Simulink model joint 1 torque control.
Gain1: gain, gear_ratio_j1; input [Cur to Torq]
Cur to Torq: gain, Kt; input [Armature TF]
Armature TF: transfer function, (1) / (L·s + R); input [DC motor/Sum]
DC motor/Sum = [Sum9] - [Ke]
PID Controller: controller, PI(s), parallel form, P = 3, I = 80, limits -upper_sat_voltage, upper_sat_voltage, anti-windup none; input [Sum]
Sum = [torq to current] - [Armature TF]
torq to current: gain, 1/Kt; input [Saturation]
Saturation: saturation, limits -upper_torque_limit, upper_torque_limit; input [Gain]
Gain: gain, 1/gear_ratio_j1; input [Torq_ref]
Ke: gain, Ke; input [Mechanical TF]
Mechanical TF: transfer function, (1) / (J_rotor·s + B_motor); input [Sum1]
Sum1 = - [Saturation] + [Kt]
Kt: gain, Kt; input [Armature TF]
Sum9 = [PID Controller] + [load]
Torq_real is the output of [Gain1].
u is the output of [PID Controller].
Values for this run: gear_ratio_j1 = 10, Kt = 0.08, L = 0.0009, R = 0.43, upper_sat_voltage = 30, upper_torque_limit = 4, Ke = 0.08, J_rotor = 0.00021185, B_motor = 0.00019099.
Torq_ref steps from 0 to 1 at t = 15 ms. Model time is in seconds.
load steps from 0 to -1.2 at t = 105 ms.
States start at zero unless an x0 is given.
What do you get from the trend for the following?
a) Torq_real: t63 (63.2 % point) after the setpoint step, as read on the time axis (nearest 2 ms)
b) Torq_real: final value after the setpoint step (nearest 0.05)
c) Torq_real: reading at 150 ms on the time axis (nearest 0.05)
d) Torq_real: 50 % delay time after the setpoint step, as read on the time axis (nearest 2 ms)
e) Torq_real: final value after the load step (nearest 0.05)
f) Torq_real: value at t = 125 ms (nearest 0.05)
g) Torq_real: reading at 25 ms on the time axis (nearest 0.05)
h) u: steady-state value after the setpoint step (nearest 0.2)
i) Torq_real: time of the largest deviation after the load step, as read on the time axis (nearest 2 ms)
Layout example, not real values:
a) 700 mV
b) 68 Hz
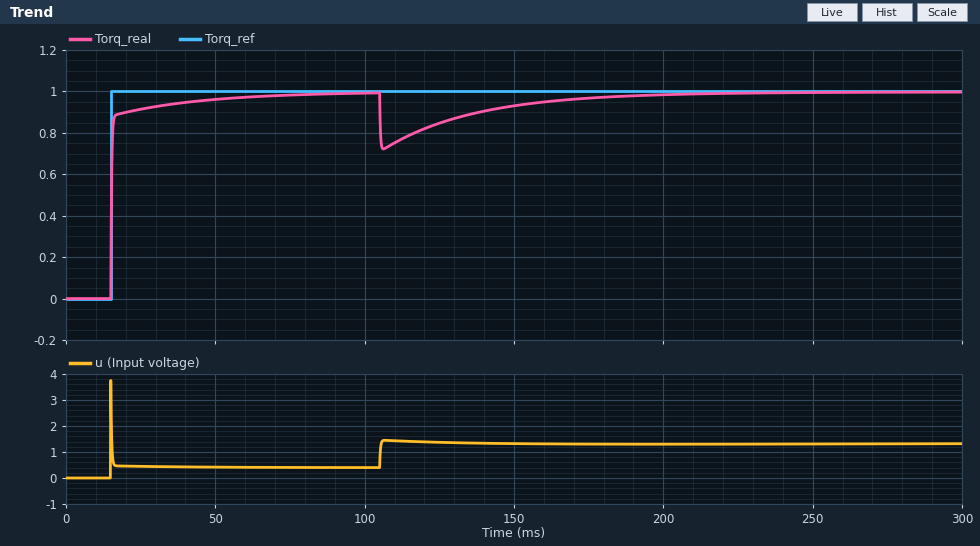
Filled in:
a) 16 ms
b) 1.00
c) 0.95
d) 16 ms
e) 1.00
f) 0.85
g) 0.90
h) 0.4
i) 106 ms
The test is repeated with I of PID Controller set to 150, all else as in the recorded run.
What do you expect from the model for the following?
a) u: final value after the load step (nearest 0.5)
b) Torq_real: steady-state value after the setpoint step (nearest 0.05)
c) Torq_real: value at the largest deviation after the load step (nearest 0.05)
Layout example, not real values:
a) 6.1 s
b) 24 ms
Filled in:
a) 1.5
b) 1.00
c) 0.75
